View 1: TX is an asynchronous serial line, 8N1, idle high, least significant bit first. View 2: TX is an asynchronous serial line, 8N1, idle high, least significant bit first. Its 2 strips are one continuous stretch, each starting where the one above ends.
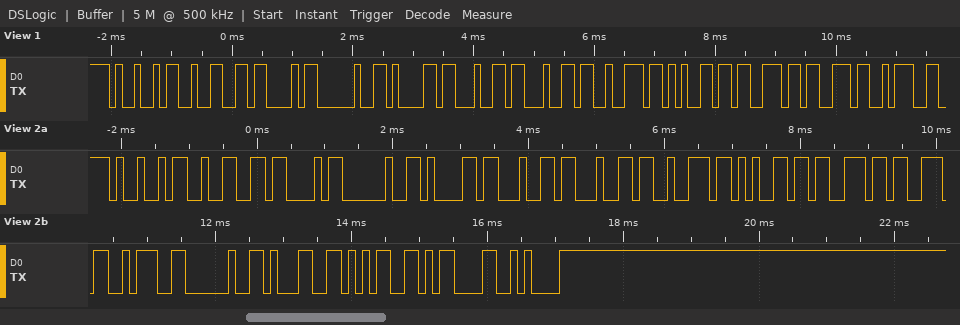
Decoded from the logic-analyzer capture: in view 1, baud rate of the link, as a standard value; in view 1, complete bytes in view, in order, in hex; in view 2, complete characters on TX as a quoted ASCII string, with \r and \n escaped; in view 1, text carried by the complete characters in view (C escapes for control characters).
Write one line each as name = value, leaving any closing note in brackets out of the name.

in view 1, baud rate of the link, as a standard value = 9600 baud
in view 1, complete bytes in view, in order, in hex = 0x49 0x32 0x43 0x20 0x61 0x64 0x64 0x72 0x65 0x73 0x73 0x3A
in view 2, complete characters on TX as a quoted ASCII string, with \r and \n escaped = "I2C address: 15\r\n"
in view 1, text carried by the complete characters in view = "I2C address:"
